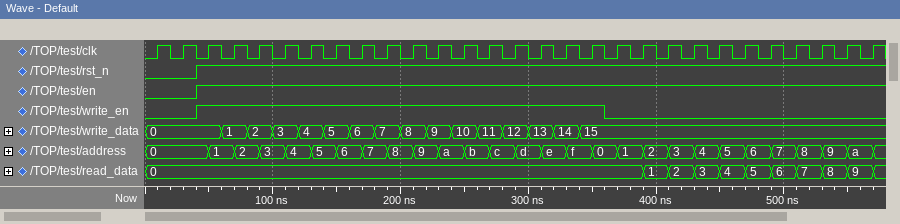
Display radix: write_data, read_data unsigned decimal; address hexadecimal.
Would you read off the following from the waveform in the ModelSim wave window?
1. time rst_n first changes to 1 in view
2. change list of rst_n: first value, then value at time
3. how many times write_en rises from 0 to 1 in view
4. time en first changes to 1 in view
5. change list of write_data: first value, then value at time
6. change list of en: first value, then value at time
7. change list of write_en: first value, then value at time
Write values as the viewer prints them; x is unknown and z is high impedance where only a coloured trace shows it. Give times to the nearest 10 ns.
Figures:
40 ns
0, 1 at 40 ns
1
40 ns
0, 1 at 60 ns, 2 at 80 ns, 3 at 100 ns, 4 at 120 ns, 5 at 140 ns, 6 at 160 ns, 7 at 180 ns, 8 at 200 ns, 9 at 220 ns, 10 at 240 ns, 11 at 260 ns, 12 at 280 ns, 13 at 300 ns, 14 at 320 ns, 15 at 340 ns
0, 1 at 40 ns
0, 1 at 40 ns, 0 at 360 ns
